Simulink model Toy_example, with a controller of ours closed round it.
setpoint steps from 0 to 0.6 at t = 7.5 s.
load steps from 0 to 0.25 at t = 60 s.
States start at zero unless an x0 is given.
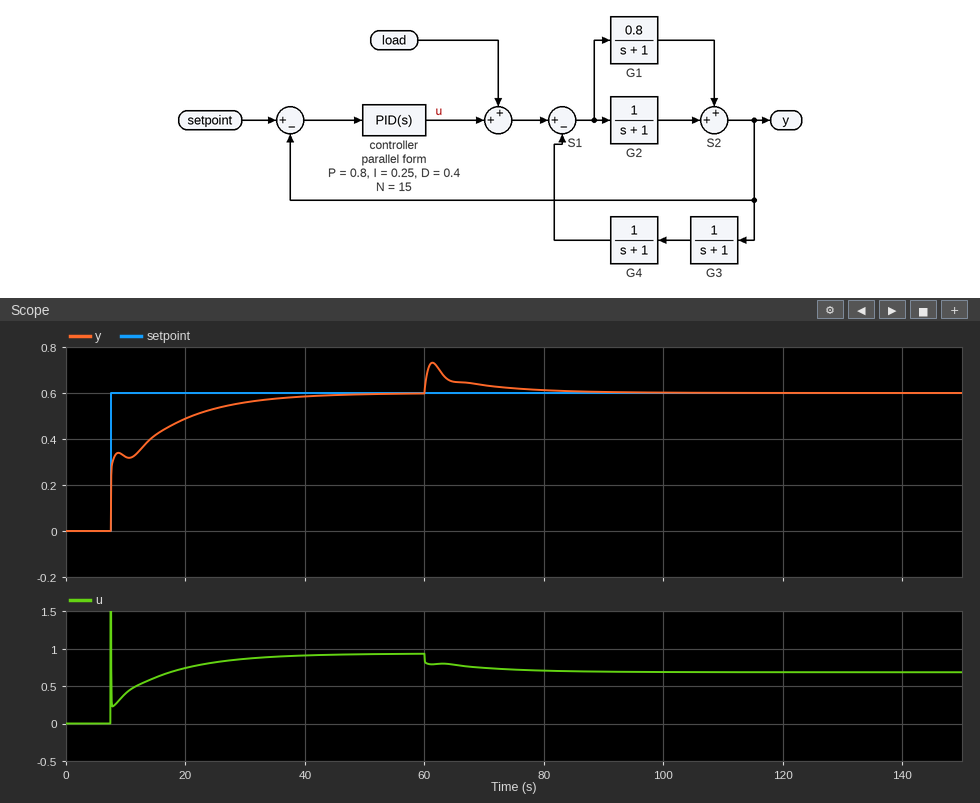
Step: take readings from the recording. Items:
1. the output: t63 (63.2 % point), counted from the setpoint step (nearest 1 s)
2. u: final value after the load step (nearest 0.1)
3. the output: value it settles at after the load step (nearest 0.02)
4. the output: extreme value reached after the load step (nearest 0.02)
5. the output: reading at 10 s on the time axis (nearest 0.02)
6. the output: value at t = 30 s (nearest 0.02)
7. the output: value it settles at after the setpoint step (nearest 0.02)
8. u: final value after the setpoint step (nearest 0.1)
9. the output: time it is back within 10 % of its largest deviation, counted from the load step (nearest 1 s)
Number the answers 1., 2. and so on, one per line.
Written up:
1. 6 s
2. 0.7
3. 0.60
4. 0.74
5. 0.32
6. 0.56
7. 0.60
8. 0.9
9. 19 s
